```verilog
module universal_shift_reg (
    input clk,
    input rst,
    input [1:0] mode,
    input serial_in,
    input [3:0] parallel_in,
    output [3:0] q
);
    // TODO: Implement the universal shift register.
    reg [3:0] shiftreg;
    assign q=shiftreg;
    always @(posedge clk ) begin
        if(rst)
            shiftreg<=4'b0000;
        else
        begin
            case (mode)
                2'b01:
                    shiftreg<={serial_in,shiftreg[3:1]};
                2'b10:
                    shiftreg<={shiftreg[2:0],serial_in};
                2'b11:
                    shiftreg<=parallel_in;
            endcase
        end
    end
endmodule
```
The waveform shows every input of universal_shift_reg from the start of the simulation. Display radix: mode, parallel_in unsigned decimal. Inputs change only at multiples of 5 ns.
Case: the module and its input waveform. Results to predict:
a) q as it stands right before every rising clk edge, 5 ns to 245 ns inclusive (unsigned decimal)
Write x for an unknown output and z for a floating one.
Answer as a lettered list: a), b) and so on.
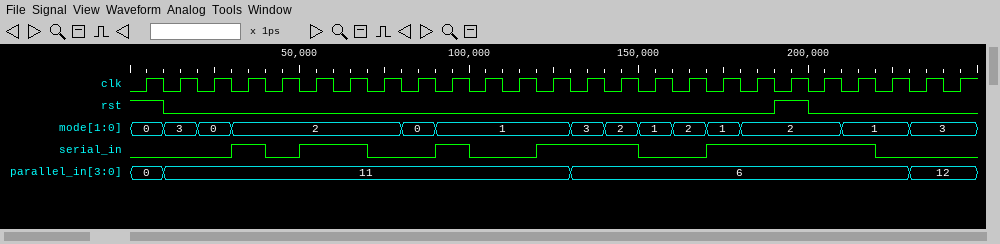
a) x, 0, 11, 11, 7, 14, 13, 11, 6, 6, 11, 5, 2, 9, 6, 13, 6, 12, 14, 13, 0, 1, 8, 4, 12
